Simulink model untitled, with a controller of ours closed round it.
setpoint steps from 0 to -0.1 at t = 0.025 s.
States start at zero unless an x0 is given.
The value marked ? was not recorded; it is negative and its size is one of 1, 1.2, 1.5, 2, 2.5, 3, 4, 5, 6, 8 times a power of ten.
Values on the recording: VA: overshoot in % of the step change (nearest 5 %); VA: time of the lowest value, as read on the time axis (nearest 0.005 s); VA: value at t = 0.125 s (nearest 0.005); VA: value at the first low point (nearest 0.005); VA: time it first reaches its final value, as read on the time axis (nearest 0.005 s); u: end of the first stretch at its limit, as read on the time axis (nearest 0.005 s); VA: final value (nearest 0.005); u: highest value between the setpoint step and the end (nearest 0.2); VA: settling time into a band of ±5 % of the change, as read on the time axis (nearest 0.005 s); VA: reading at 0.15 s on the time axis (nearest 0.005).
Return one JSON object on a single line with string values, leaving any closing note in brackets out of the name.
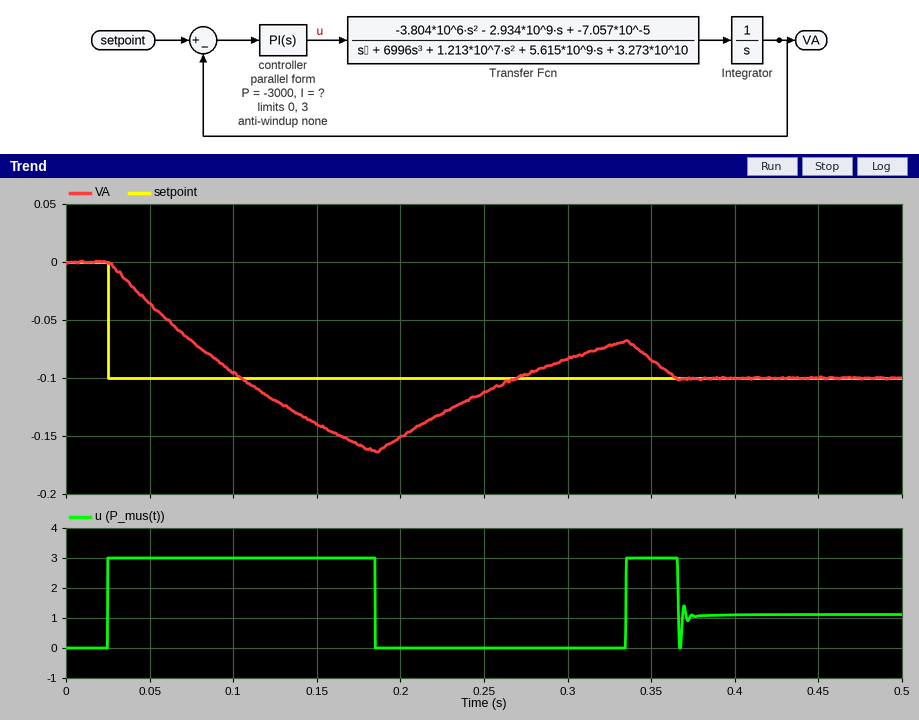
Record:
{"VA: overshoot in % of the step change": "65 %", "VA: time of the lowest value, as read on the time axis": "0.185 s", "VA: value at t = 0.125 s": "-0.120", "VA: value at the first low point": "-0.165", "VA: time it first reaches its final value, as read on the time axis": "0.105 s", "u: end of the first stretch at its limit, as read on the time axis": "0.185 s", "VA: final value": "-0.100", "u: highest value between the setpoint step and the end": "3.0", "VA: settling time into a band of ±5 % of the change, as read on the time axis": "0.360 s", "VA: reading at 0.15 s on the time axis": "-0.140"}
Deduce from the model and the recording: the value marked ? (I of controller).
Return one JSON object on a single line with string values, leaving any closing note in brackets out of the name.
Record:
{"the value marked ?": "-200000"}
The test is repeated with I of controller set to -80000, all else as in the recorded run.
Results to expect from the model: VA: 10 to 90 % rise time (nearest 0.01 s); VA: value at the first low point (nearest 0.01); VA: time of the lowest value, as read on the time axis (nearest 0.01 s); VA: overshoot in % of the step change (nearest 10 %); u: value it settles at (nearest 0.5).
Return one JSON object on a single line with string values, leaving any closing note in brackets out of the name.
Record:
{"VA: 10 to 90 % rise time": "0.06 s", "VA: value at the first low point": "-0.15", "VA: time of the lowest value, as read on the time axis": "0.17 s", "VA: overshoot in % of the step change": "50 %", "u: value it settles at": "1.0"}
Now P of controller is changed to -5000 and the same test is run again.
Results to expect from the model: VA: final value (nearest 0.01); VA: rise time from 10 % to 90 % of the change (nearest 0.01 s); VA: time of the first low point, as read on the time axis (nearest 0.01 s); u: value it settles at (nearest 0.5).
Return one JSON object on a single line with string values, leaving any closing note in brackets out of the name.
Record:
{"VA: final value": "-0.10", "VA: rise time from 10 % to 90 % of the change": "0.06 s", "VA: time of the first low point, as read on the time axis": "0.18 s", "u: value it settles at": "1.0"}
